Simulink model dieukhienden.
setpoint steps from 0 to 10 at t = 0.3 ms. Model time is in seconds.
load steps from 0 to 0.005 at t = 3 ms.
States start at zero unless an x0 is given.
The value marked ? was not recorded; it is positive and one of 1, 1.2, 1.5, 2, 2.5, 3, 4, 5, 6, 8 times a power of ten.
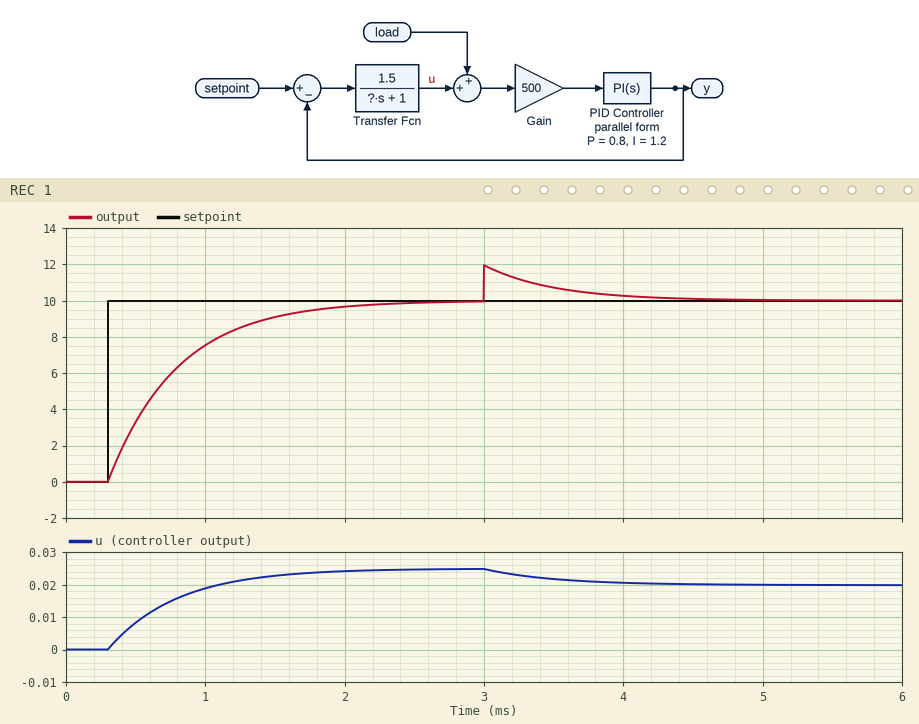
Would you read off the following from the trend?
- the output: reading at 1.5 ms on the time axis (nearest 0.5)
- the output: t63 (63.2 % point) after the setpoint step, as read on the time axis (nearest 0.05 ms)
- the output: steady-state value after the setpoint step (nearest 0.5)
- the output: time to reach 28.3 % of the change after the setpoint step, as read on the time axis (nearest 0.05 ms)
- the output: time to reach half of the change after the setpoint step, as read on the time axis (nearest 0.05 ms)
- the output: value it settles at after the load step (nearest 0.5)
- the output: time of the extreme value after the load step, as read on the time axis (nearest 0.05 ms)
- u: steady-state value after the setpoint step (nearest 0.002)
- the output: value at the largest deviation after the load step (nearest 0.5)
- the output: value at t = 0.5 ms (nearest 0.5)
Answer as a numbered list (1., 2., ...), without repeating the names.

1. 9.0
2. 0.80 ms
3. 10.0
4. 0.45 ms
5. 0.65 ms
6. 10.0
7. 3.00 ms
8. 0.024
9. 12.0
10. 3.5
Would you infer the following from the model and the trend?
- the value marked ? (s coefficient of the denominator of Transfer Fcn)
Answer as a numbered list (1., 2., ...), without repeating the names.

1. 0.3
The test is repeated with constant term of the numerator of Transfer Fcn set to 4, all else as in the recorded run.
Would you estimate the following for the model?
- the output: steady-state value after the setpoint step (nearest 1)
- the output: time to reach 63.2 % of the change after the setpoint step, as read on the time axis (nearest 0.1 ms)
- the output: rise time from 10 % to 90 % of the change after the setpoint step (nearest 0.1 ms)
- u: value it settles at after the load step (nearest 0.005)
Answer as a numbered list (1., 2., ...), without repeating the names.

1. 10
2. 0.5 ms
3. 0.4 ms
4. 0.020
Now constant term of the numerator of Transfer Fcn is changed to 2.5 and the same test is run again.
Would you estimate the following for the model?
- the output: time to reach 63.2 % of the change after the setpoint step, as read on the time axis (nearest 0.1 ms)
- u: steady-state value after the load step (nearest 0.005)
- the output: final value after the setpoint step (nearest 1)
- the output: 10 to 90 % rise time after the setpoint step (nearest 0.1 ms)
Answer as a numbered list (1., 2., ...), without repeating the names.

1. 0.6 ms
2. 0.020
3. 10
4. 0.7 ms
